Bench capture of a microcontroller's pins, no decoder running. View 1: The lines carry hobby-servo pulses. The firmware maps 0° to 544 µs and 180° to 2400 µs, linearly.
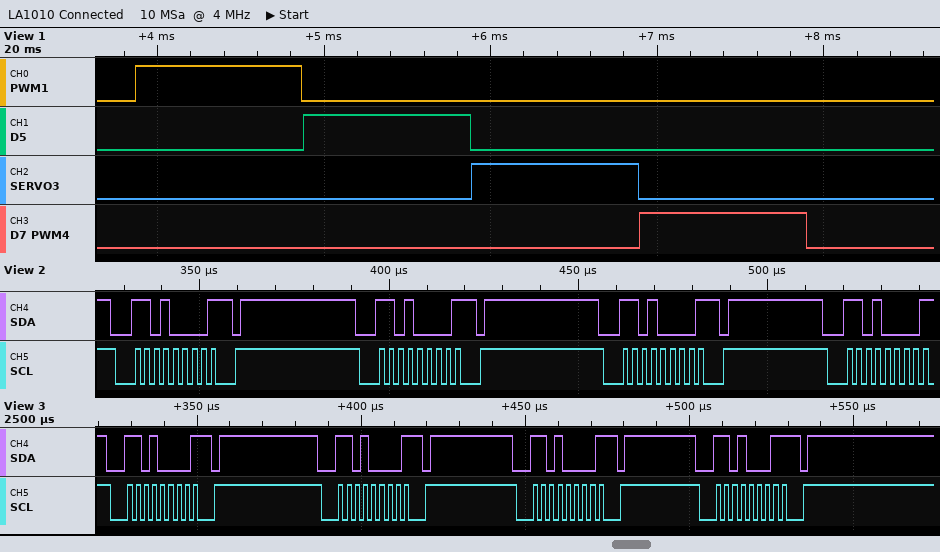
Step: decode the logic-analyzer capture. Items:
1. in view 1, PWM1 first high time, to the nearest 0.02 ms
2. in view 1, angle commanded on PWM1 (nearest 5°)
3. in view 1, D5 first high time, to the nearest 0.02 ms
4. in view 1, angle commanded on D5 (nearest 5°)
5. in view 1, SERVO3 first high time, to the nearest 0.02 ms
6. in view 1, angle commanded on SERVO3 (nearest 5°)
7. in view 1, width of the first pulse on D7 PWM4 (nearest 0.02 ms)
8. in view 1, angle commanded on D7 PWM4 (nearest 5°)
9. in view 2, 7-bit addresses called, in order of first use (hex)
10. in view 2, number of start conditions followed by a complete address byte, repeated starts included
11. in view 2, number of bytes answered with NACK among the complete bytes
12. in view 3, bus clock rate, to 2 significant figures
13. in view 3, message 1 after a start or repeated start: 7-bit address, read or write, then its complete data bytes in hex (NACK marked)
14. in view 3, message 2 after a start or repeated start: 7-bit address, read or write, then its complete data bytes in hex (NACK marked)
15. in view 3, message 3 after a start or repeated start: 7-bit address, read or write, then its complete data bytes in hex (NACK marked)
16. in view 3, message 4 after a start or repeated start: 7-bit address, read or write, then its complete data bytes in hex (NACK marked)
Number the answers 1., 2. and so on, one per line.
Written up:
1. 1.00 ms
2. 45°
3. 1.00 ms
4. 45°
5. 1.00 ms
6. 45°
7. 1.00 ms
8. 45°
9. 0x68
10. 4
11. 4
12. 400 kHz
13. 0x68 write NACK
14. 0x68 write NACK
15. 0x68 write NACK
16. 0x68 read NACK
